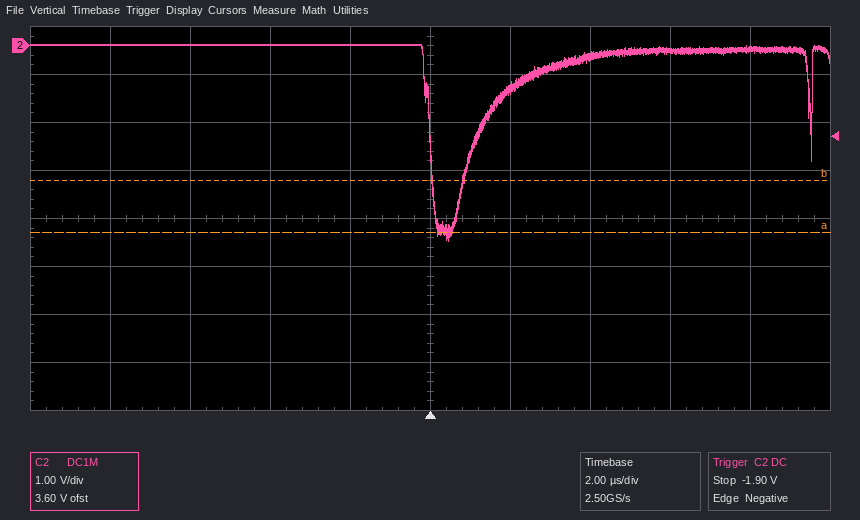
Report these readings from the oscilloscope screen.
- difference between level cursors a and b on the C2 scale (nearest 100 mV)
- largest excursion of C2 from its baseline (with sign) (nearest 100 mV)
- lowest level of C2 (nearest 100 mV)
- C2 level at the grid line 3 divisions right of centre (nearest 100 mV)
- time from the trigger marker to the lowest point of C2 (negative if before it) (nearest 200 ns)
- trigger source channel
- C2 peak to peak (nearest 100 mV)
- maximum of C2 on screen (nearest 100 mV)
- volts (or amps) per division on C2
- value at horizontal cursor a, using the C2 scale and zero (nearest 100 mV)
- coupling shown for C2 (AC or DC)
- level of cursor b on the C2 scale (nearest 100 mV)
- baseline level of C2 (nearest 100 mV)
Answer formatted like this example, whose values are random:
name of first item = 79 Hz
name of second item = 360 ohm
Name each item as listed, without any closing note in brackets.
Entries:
difference between level cursors a and b on the C2 scale = 1.1 V
largest excursion of C2 from its baseline (with sign) = -4.1 V
lowest level of C2 = -4.1 V
C2 level at the grid line 3 divisions right of centre = -100 mV
time from the trigger marker to the lowest point of C2 (negative if before it) = +400 ns
trigger source channel = C2
C2 peak to peak = 4.1 V
maximum of C2 on screen = 0.0 V
volts (or amps) per division on C2 = 1 V
value at horizontal cursor a, using the C2 scale and zero = -3.9 V
coupling shown for C2 = DC
level of cursor b on the C2 scale = -2.8 V
baseline level of C2 = 0.0 V
